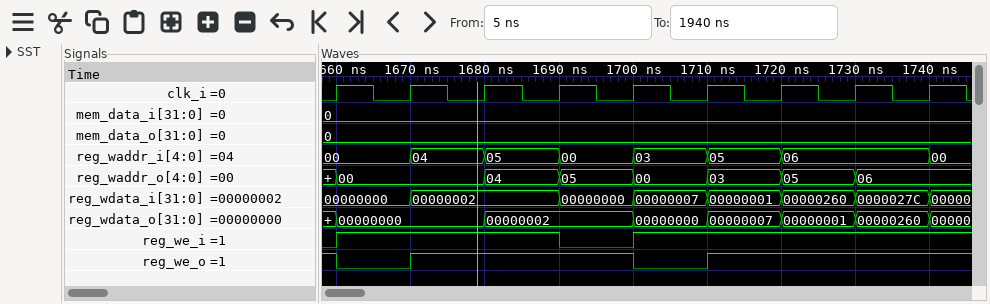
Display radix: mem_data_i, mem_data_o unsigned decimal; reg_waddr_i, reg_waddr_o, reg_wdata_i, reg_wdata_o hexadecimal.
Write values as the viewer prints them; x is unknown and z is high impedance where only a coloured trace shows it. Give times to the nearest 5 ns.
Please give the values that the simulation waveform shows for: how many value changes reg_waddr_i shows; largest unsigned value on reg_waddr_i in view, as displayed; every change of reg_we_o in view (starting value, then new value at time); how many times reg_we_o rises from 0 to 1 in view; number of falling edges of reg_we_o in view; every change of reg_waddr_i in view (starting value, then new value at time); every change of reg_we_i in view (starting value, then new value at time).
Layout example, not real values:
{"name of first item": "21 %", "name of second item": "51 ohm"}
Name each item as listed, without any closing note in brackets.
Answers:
{"how many value changes reg_waddr_i shows": "7", "largest unsigned value on reg_waddr_i in view, as displayed": "06", "every change of reg_we_o in view": "1, 0 at 1660 ns, 1 at 1670 ns, 0 at 1700 ns, 1 at 1710 ns", "how many times reg_we_o rises from 0 to 1 in view": "2", "number of falling edges of reg_we_o in view": "2", "every change of reg_waddr_i in view": "00, 04 at 1670 ns, 05 at 1680 ns, 00 at 1690 ns, 03 at 1700 ns, 05 at 1710 ns, 06 at 1720 ns, 00 at 1740 ns", "every change of reg_we_i in view": "0, 1 at 1660 ns, 0 at 1690 ns, 1 at 1700 ns"}
